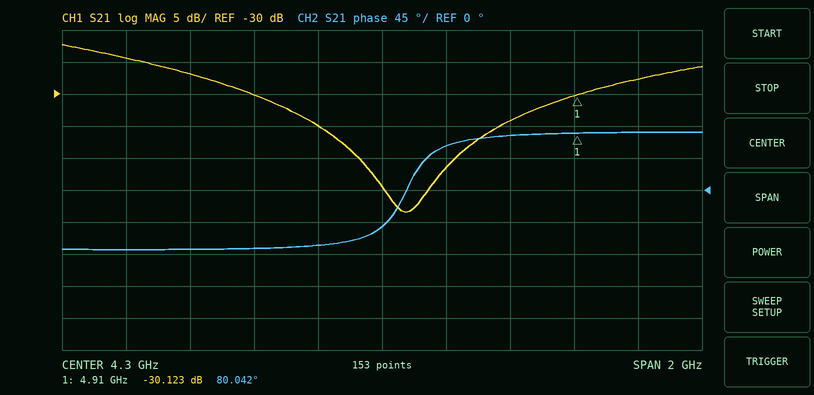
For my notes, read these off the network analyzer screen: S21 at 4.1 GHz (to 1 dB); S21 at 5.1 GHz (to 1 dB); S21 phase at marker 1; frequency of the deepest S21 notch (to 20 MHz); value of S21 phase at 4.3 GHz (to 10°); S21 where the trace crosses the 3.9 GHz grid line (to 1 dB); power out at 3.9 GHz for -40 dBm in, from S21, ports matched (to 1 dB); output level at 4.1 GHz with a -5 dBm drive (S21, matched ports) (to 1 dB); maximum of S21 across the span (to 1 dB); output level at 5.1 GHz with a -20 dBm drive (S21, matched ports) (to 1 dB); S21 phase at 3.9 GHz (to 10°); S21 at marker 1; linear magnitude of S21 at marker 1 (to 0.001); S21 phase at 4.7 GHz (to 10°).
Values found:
-35 dB
-28 dB
80.042°
4.38 GHz
-50°
-30 dB
-70 dBm
-40 dBm
-22 dB
-48 dBm
-80°
-30.123 dB
0.031
80°
